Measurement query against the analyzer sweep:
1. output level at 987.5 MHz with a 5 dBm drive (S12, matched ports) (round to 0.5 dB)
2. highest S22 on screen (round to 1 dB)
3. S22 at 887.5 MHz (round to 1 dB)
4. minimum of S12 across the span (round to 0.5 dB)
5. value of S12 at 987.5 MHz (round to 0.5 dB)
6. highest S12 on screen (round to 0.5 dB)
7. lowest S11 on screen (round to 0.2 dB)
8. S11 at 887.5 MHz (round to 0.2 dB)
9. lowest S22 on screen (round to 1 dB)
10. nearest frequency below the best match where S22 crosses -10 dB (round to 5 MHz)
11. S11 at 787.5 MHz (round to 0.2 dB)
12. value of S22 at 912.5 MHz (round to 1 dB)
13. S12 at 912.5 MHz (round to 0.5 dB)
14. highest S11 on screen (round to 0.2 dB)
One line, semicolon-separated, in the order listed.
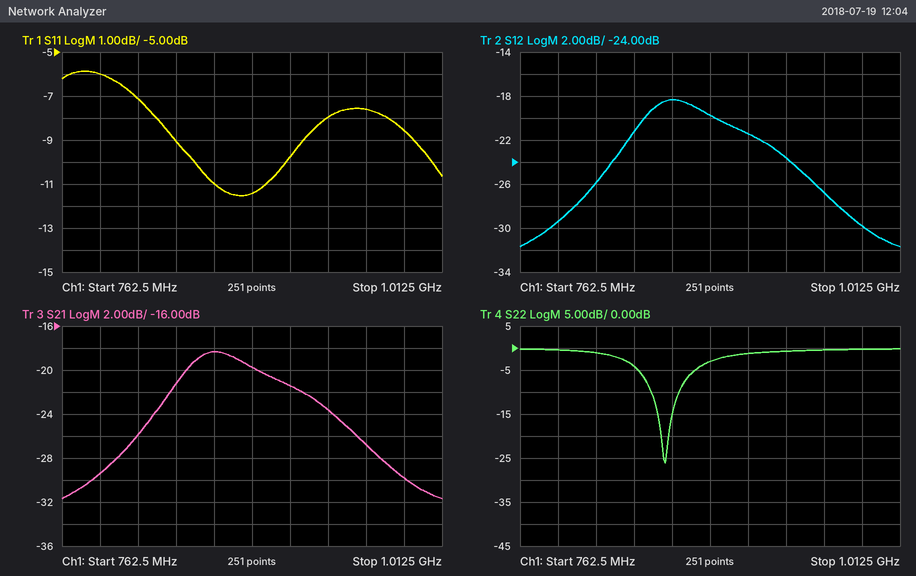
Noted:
-25.0 dBm; 0 dB; -3 dB; -31.5 dB; -30.0 dB; -18.5 dB; -11.6 dB; -11.4 dB; -26 dB; 850 MHz; -6.0 dB; -1 dB; -21.5 dB; -5.8 dB
